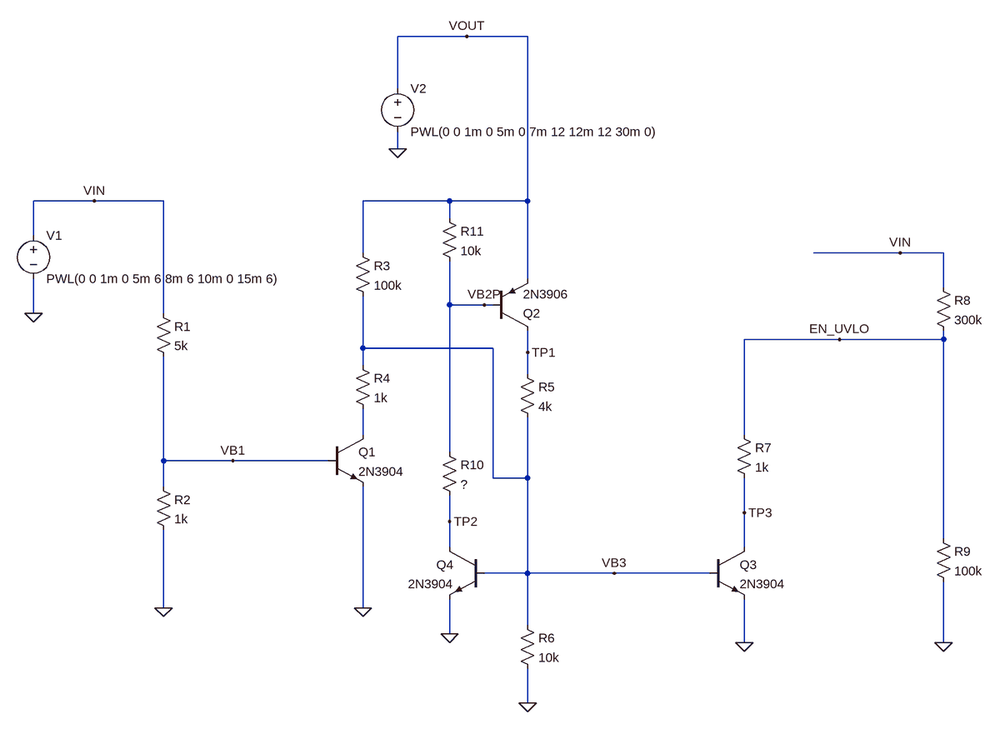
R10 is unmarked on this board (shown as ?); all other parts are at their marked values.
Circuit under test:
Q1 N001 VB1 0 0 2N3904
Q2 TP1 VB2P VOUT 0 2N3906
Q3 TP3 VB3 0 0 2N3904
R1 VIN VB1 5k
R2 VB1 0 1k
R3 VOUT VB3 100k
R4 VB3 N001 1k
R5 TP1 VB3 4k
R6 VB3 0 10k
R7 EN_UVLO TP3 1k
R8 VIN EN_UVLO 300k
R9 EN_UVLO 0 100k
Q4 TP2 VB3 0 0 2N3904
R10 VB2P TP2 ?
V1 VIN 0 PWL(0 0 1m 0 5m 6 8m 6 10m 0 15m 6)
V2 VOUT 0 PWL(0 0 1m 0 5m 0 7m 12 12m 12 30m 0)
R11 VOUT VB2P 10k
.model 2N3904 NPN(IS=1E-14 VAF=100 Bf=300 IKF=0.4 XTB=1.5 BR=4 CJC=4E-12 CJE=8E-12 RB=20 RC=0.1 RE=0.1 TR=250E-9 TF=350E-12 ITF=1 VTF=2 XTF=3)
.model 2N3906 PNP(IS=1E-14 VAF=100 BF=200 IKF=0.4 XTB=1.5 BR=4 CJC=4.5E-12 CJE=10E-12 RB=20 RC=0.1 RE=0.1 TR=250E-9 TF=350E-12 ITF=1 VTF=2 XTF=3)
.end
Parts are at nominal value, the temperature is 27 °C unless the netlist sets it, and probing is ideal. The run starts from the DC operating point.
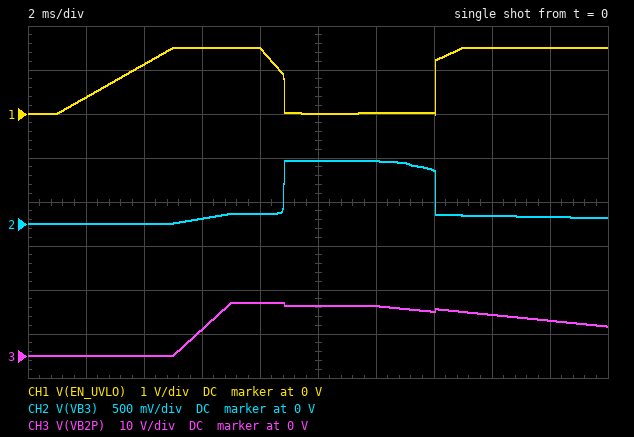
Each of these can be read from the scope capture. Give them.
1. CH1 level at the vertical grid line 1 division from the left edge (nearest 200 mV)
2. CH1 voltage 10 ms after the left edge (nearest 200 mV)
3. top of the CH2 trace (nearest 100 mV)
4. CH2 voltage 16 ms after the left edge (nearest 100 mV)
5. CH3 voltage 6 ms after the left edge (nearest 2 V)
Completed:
400 mV
0 V
700 mV
100 mV
6 V
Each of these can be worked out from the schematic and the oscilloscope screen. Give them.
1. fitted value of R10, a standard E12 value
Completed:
150 kΩ
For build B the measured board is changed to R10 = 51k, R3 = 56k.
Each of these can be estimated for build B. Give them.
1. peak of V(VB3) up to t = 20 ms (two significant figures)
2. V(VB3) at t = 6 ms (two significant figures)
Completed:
740 mV
100 mV
